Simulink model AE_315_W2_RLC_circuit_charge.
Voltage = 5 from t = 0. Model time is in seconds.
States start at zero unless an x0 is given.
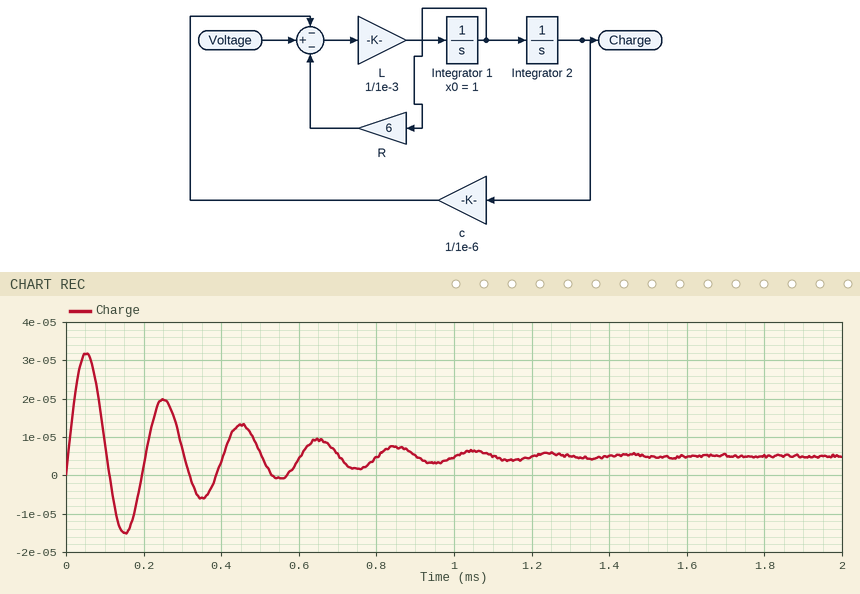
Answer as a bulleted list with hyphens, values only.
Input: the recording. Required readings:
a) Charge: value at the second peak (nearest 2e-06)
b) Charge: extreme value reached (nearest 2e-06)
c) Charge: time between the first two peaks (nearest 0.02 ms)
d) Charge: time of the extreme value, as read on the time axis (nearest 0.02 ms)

- 0.000020
- 0.000032
- 0.20 ms
- 0.06 ms
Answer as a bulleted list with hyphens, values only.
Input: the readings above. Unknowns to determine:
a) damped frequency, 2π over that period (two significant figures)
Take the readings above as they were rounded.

- 31 rad/ms
